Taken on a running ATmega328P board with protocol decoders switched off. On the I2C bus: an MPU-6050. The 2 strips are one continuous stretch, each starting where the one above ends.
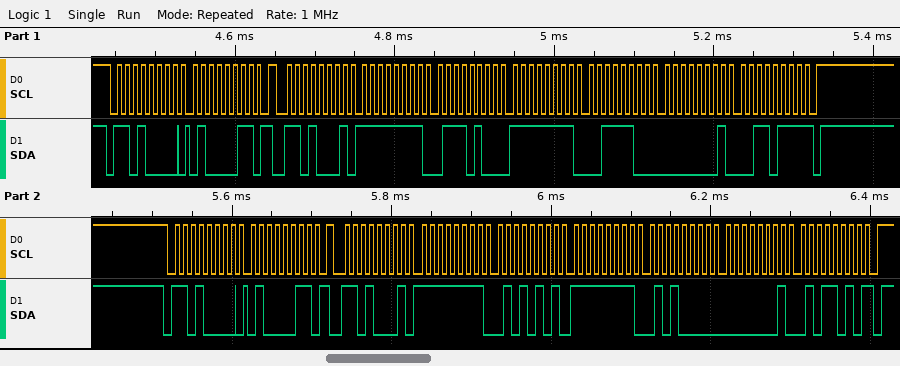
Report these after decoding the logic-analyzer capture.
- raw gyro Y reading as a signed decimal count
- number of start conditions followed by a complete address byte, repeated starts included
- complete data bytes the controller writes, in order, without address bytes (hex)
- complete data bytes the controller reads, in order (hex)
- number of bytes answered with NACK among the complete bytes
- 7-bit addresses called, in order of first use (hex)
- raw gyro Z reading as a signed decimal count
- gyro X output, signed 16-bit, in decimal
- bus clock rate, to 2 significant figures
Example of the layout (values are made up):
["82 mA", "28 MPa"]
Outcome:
["-196", "4", "43 43", "FF 74 FF 3C 01 37 FF 55 FF 50 01 5A", "2", "0x68", "311", "-140", "100 kHz"]
